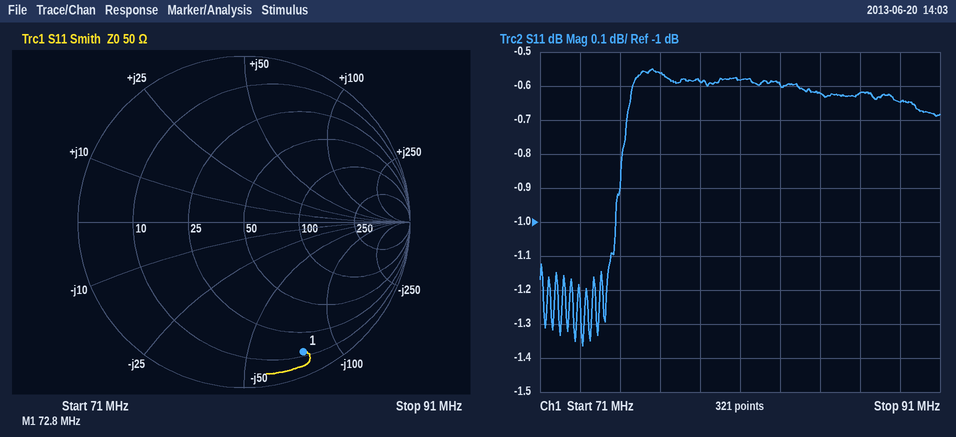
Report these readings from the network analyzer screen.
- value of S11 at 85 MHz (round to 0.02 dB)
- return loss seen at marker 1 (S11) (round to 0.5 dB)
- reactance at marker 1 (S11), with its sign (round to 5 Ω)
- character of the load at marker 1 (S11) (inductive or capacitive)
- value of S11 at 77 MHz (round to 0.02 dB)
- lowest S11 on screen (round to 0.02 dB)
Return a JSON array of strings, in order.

["-0.62 dB", "1.5 dB", "-75 Ω", "capacitive", "-0.56 dB", "-1.36 dB"]
